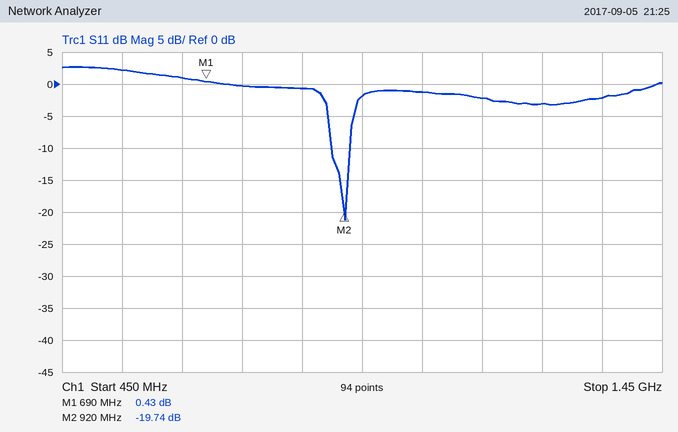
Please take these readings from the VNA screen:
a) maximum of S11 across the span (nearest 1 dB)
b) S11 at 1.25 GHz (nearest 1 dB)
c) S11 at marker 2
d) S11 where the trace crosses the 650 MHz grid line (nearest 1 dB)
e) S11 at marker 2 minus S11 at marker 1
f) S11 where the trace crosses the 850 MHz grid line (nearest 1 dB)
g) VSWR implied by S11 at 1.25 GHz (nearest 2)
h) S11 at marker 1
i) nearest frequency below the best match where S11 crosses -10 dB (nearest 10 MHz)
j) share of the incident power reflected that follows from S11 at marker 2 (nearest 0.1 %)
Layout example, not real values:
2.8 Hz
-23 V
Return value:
3 dB
-3 dB
-19.74 dB
1 dB
-20.17 dB
-1 dB
6
0.43 dB
900 MHz
1.1 %
